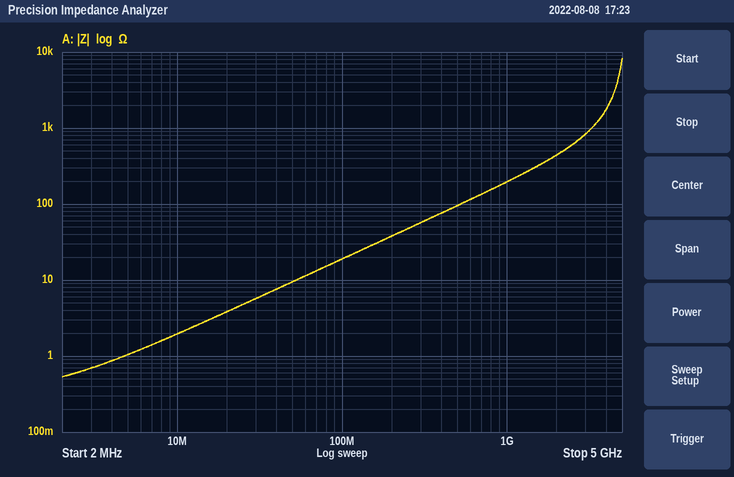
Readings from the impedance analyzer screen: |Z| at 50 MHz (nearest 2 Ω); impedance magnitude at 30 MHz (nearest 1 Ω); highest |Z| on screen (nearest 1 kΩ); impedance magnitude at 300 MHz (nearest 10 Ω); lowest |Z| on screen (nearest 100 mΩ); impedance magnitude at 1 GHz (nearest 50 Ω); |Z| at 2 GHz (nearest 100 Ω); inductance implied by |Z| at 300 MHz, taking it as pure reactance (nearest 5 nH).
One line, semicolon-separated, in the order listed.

10 Ω; 6 Ω; 8 kΩ; 60 Ω; 500 mΩ; 200 Ω; 400 Ω; 30 nH
